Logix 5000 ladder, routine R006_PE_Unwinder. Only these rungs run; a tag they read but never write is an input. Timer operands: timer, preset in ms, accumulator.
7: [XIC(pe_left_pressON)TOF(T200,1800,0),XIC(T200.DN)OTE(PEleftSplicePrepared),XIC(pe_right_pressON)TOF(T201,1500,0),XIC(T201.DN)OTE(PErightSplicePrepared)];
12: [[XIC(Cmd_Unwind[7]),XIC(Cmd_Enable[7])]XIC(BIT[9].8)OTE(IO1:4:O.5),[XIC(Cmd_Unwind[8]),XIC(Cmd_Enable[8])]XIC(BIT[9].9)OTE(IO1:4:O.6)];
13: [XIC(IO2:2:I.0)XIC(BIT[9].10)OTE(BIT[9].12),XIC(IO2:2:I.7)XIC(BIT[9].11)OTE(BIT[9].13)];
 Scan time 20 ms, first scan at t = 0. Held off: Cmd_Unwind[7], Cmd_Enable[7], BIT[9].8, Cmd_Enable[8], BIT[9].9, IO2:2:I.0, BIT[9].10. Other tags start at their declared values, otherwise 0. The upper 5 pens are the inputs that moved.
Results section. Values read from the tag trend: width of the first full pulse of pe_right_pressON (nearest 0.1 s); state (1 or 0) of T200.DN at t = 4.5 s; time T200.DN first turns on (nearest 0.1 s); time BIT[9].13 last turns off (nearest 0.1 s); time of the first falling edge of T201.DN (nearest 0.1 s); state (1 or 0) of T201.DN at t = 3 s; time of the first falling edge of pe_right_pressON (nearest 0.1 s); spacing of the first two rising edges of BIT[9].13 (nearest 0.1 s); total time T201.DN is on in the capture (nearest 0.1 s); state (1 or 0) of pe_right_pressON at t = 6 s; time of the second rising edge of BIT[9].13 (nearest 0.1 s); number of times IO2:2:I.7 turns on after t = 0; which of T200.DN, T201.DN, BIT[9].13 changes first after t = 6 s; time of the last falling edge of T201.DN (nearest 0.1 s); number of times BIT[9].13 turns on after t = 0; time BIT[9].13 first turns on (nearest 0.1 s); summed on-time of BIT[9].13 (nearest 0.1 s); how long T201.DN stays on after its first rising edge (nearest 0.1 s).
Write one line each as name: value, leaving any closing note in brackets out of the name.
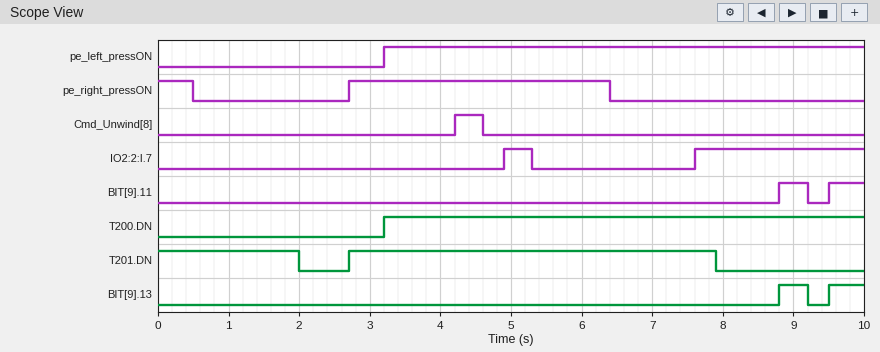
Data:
width of the first full pulse of pe_right_pressON: 3.7 s
state (1 or 0) of T200.DN at t = 4.5 s: 1
time T200.DN first turns on: 3.2 s
time BIT[9].13 last turns off: 9.2 s
time of the first falling edge of T201.DN: 2.0 s
state (1 or 0) of T201.DN at t = 3 s: 1
time of the first falling edge of pe_right_pressON: 0.5 s
spacing of the first two rising edges of BIT[9].13: 0.7 s
total time T201.DN is on in the capture: 7.2 s
state (1 or 0) of pe_right_pressON at t = 6 s: 1
time of the second rising edge of BIT[9].13: 9.5 s
number of times IO2:2:I.7 turns on after t = 0: 2
which of T200.DN, T201.DN, BIT[9].13 changes first after t = 6 s: T201.DN
time of the last falling edge of T201.DN: 7.9 s
number of times BIT[9].13 turns on after t = 0: 2
time BIT[9].13 first turns on: 8.8 s
summed on-time of BIT[9].13: 0.9 s
how long T201.DN stays on after its first rising edge: 5.2 s
